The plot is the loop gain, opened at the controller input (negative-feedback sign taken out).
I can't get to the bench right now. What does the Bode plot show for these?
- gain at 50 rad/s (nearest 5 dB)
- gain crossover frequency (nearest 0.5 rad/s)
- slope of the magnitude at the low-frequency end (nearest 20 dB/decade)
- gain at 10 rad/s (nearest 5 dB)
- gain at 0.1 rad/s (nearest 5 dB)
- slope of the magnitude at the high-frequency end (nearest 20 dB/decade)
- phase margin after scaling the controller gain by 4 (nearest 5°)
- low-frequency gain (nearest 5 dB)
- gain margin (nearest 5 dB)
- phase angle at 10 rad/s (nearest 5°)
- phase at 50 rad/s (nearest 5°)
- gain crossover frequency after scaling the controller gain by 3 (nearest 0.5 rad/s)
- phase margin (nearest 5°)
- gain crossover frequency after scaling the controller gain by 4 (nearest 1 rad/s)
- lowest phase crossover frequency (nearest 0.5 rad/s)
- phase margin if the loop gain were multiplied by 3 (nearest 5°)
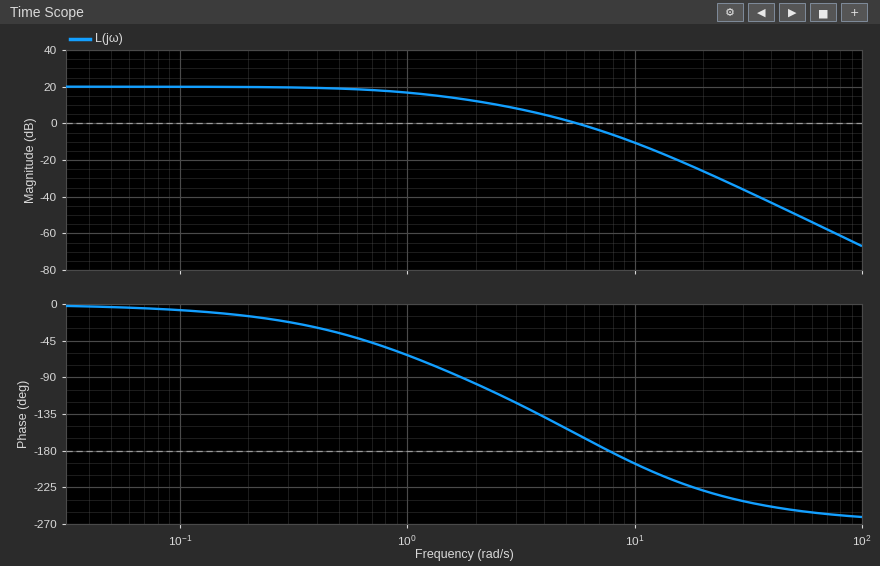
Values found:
-50 dB
5.5 rad/s
0 dB/decade
-10 dB
20 dB
-60 dB/decade
-20°
20 dB
5 dB
-195°
-255°
9.5 rad/s
20°
11 rad/s
7.5 rad/s
-15°
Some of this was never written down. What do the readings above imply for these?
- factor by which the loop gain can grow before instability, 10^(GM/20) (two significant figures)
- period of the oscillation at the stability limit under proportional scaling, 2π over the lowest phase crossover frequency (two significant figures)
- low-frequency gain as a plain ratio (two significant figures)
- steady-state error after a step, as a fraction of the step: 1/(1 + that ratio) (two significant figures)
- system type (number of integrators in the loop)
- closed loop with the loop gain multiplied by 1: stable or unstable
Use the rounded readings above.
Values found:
1.8
0.84 s
10
0.091
0
stable
